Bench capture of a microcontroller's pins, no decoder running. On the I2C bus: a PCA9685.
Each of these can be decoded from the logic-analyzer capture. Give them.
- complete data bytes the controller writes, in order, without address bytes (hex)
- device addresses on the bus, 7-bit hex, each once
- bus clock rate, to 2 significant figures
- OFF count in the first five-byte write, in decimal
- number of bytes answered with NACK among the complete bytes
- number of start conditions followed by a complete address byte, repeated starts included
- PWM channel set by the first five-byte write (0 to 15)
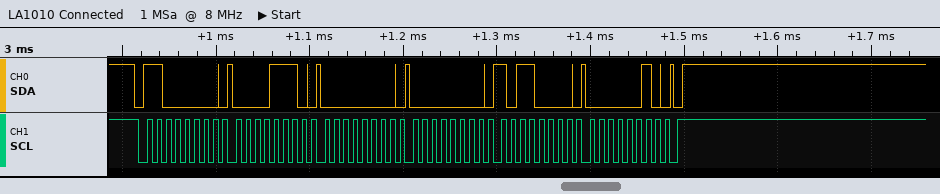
0E 00 00 B0 02
0x60
100 kHz
688
0
1
2
